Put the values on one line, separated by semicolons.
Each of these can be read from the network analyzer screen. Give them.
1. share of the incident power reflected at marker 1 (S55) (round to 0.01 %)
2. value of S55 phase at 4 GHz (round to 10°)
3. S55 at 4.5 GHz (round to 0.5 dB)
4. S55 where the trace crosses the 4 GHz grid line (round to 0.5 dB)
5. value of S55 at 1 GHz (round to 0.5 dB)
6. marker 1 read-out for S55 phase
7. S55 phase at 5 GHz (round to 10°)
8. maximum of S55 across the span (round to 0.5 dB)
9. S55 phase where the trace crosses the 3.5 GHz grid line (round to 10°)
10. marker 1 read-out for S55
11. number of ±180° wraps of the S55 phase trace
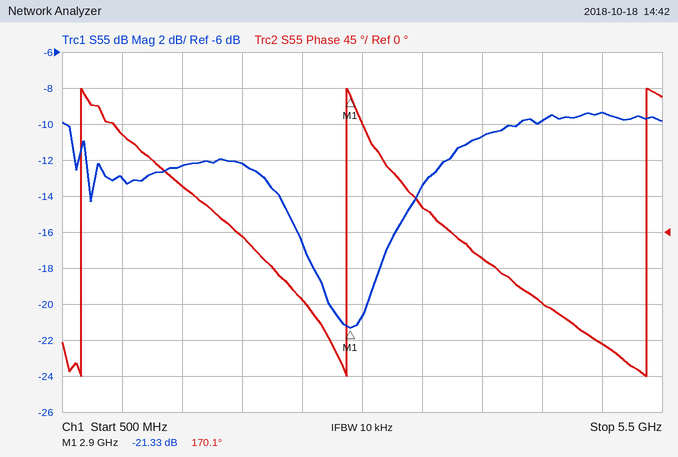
0.74 %; -30°; -10.0 dB; -10.5 dB; -13.0 dB; 170.1°; -140°; -9.5 dB; 30°; -21.33 dB; 3
